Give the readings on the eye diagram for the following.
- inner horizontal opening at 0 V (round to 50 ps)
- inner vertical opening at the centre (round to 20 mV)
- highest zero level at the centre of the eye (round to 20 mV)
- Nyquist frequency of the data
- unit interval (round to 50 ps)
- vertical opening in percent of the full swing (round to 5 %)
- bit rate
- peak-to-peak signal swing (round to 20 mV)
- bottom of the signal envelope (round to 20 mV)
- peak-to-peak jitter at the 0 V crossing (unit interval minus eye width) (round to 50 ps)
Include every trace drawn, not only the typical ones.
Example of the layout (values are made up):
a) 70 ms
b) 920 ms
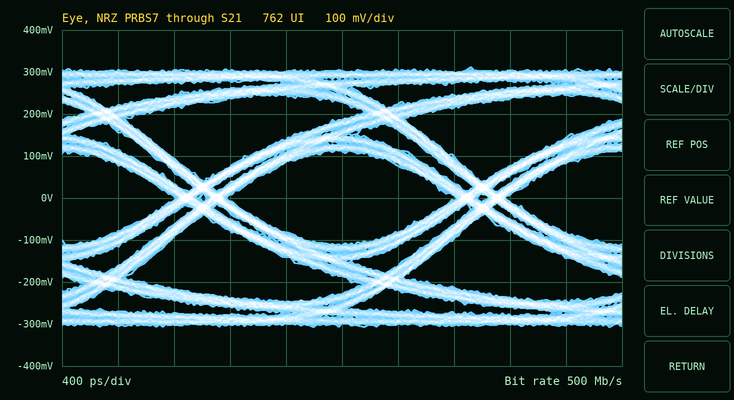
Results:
a) 1.65 ns
b) 220 mV
c) -120 mV
d) 250 MHz
e) 2.00 ns
f) 35 %
g) 500 Mb/s
h) 620 mV
i) -300 mV
j) 350 ps
